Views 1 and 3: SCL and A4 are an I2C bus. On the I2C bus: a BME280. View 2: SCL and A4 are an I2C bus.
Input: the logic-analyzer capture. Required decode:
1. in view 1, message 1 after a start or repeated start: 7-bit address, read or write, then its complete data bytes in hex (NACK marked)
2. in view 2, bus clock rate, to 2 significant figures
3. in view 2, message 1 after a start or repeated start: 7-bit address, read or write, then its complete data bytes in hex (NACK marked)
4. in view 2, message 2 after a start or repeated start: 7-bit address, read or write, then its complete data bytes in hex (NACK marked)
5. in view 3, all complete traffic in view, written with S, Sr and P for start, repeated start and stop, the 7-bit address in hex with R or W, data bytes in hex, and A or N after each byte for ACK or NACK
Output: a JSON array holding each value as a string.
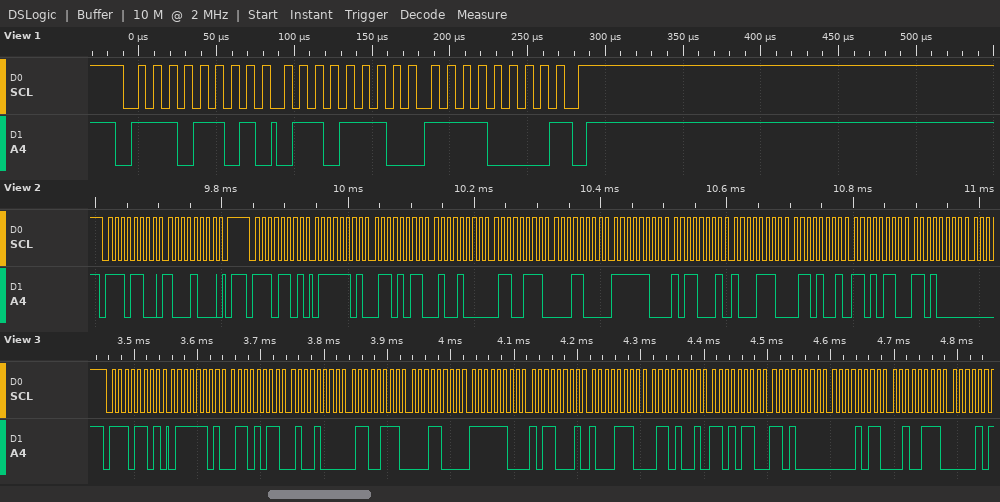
["0x76 read: 6E F0 NACK", "100 kHz", "0x76 write: 88", "0x76 read: 7D 6B 48 67 18 FC B1 8E 69 D6 D0", "S 76R A 7D A 6B A 48 A 67 A 18 A FC A B1 A 8E A 69 A D6 A D0 A 0B A 27 A"]
